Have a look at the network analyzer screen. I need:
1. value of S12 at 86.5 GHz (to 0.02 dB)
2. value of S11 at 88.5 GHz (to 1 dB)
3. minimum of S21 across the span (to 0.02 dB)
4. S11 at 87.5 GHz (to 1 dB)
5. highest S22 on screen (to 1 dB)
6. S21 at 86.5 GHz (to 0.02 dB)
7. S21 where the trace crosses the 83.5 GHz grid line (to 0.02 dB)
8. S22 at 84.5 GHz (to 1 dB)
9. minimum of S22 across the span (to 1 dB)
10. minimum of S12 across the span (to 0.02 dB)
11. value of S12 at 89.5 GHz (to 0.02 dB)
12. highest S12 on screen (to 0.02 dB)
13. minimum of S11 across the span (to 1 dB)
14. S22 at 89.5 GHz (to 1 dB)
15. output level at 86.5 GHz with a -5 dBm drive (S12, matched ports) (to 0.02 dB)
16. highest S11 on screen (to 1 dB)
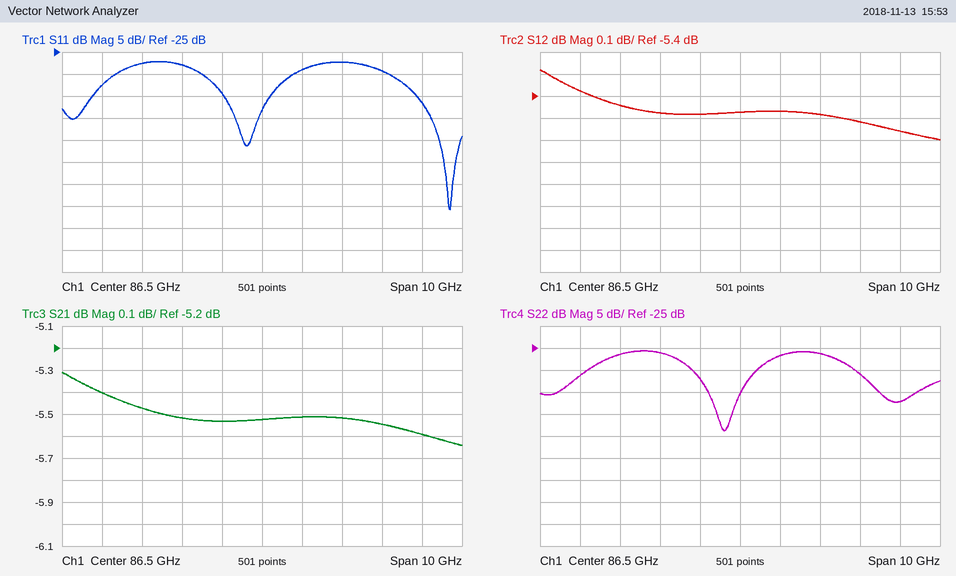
-5.48 dB
-27 dB
-5.64 dB
-29 dB
-26 dB
-5.52 dB
-5.48 dB
-26 dB
-44 dB
-5.60 dB
-5.52 dB
-5.28 dB
-61 dB
-31 dB
-10.48 dBm
-27 dB
